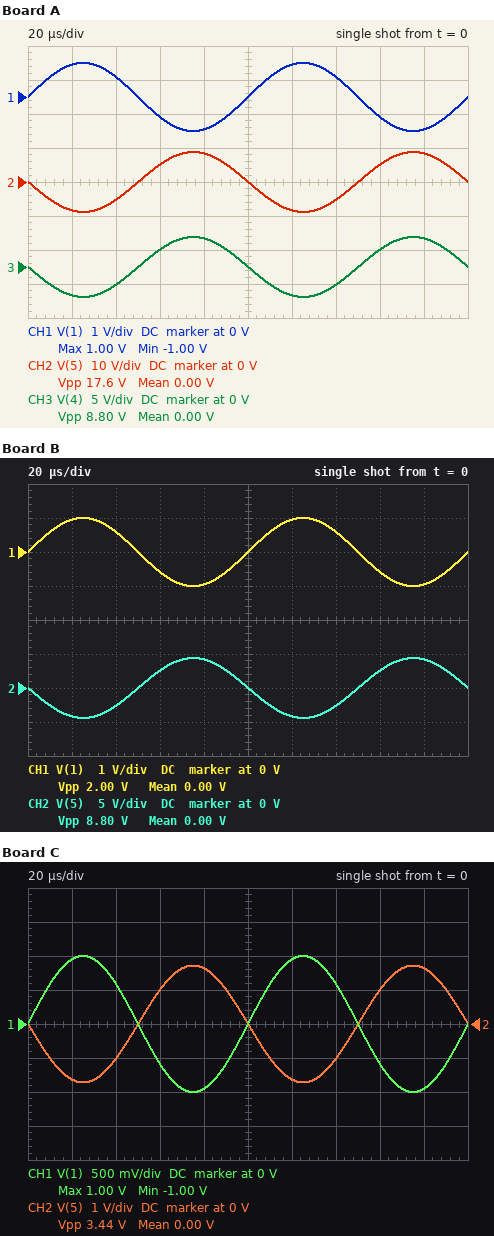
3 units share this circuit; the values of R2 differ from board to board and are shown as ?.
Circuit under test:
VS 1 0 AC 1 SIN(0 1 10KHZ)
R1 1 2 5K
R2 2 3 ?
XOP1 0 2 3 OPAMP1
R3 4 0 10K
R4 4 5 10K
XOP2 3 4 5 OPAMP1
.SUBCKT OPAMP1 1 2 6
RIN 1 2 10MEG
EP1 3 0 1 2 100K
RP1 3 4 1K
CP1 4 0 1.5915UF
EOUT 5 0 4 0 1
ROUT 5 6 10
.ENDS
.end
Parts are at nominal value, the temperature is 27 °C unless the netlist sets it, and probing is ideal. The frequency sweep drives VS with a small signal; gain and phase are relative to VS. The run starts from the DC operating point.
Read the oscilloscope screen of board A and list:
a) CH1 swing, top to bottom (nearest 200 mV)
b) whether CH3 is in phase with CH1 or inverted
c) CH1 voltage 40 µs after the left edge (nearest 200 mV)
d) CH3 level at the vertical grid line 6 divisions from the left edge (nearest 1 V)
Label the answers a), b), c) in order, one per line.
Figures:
a) 2.0 V
b) inverted
c) 600 mV
d) -4 V
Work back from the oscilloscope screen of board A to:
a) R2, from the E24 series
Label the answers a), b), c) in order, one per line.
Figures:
a) 22 kΩ
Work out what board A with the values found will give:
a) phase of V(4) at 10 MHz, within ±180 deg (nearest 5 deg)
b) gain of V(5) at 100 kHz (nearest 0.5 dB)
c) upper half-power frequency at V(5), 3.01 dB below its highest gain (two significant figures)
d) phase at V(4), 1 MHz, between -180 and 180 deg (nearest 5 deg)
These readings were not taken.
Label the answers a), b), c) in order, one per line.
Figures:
a) 35 deg
b) 19.0 dB
c) 1.7 MHz
d) 140 deg
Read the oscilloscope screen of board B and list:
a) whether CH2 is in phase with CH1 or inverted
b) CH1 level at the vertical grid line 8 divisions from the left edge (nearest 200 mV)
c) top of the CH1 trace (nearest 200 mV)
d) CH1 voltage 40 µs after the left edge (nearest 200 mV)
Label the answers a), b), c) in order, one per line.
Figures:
a) inverted
b) -600 mV
c) 1.0 V
d) 600 mV
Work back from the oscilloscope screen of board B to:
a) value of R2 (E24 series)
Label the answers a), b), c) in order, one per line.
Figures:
a) 11 kΩ
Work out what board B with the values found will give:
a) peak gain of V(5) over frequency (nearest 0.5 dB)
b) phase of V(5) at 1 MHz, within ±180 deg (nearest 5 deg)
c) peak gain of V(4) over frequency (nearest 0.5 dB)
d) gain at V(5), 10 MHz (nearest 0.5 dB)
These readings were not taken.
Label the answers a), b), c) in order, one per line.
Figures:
a) 13.0 dB
b) 150 deg
c) 7.0 dB
d) -4.5 dB
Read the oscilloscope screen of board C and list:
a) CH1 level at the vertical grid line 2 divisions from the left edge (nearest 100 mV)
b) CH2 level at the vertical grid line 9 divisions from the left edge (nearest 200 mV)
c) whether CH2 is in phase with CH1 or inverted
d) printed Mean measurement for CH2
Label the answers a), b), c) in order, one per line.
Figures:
a) 600 mV
b) 1.6 V
c) inverted
d) 0.00 V
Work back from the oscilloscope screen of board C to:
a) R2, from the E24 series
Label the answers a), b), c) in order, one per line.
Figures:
a) 4.3 kΩ
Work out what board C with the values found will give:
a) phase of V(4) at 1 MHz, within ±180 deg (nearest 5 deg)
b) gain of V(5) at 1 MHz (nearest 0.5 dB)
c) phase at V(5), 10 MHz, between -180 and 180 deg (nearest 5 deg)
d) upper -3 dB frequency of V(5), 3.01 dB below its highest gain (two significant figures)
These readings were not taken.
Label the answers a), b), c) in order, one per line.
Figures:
a) 160 deg
b) 4.5 dB
c) 55 deg
d) 3.3 MHz
